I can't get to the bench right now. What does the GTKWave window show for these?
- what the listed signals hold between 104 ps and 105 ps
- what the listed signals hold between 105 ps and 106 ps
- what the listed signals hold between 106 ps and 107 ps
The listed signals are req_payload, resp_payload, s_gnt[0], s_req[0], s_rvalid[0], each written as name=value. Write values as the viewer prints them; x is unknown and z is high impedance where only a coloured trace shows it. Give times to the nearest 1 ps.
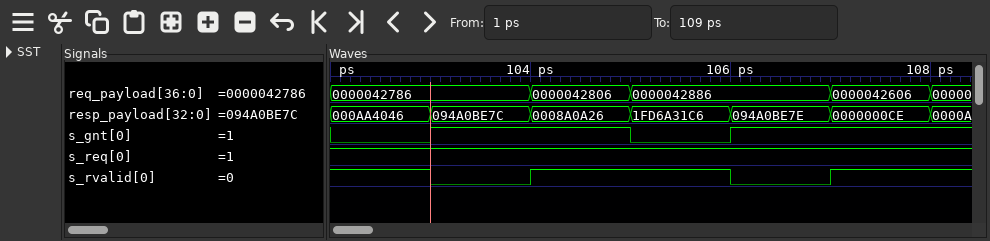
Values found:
req_payload=0000042806, resp_payload=0008A0A26, s_gnt[0]=1, s_req[0]=1, s_rvalid[0]=1
req_payload=0000042886, resp_payload=1FD6A31C6, s_gnt[0]=0, s_req[0]=1, s_rvalid[0]=1
req_payload=0000042886, resp_payload=094A0BE7E, s_gnt[0]=1, s_req[0]=1, s_rvalid[0]=0
